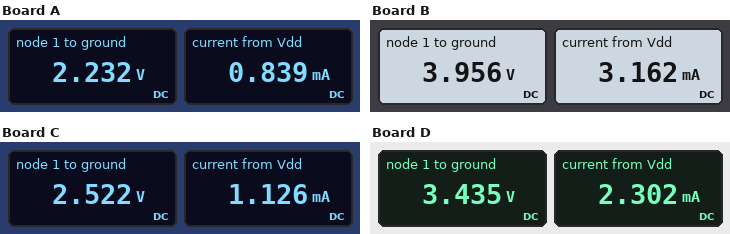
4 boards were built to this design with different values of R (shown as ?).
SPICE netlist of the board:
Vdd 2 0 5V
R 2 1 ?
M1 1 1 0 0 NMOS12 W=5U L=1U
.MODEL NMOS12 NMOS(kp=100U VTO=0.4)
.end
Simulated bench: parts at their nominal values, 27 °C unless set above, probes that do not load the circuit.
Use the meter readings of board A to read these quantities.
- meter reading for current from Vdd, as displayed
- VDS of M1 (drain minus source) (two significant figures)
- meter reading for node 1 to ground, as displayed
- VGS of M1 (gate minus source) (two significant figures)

0.839 mA
2.2 V
2.232 V
2.2 V
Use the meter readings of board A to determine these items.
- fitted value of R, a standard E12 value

3.3 kΩ
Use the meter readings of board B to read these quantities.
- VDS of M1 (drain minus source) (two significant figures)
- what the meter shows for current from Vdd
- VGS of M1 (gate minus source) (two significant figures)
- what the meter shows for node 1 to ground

4.0 V
3.162 mA
4.0 V
3.956 V
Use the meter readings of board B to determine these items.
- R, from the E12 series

330 Ω
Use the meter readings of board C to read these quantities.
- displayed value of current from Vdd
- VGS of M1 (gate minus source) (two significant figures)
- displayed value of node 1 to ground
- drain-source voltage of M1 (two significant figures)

1.126 mA
2.5 V
2.522 V
2.5 V
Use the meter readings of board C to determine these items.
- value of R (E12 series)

2.2 kΩ
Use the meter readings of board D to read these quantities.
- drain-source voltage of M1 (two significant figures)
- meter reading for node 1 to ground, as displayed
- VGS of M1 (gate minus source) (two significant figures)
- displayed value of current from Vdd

3.4 V
3.435 V
3.4 V
2.302 mA
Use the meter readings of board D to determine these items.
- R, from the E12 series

680 Ω
